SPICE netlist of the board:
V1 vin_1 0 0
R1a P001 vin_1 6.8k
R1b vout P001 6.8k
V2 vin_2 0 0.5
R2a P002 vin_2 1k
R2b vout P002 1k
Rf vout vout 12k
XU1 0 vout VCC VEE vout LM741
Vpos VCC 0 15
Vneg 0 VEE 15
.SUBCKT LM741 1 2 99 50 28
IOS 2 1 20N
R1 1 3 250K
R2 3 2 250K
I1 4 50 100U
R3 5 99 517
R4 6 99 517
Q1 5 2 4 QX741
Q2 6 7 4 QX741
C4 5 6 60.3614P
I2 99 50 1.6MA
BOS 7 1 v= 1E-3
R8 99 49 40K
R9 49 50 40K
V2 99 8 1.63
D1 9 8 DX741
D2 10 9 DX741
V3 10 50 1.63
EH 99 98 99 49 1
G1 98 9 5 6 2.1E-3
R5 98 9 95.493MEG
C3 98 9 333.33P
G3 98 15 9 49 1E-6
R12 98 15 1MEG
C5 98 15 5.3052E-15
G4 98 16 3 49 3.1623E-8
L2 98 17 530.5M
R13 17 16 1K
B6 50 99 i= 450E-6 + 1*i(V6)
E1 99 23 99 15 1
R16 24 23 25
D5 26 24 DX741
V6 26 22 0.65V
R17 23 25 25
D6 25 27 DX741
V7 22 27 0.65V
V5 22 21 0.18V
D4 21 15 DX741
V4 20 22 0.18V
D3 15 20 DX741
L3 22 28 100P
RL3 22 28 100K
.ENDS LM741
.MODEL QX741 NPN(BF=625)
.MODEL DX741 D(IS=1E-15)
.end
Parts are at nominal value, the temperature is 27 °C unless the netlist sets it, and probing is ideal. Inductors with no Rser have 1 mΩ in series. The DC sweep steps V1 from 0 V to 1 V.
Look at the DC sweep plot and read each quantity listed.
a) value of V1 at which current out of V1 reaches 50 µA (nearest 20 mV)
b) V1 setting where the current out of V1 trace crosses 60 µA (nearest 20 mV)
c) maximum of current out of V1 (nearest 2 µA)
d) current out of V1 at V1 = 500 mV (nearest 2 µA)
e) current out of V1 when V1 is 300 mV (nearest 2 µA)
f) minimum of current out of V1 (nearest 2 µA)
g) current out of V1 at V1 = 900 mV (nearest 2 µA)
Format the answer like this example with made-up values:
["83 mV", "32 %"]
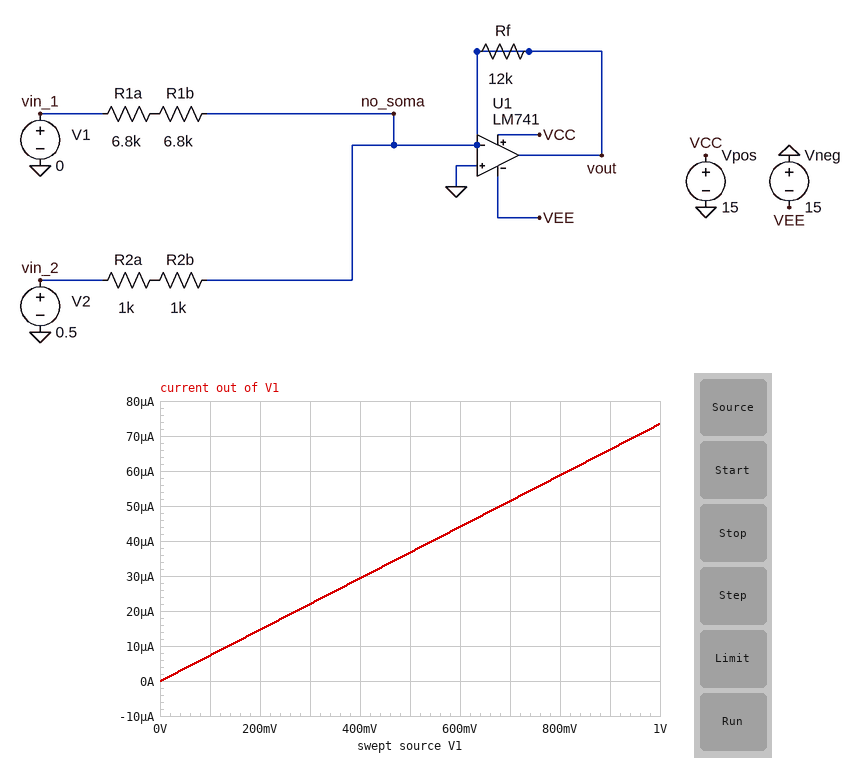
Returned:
["680 mV", "820 mV", "74 µA", "36 µA", "22 µA", "0 A", "66 µA"]
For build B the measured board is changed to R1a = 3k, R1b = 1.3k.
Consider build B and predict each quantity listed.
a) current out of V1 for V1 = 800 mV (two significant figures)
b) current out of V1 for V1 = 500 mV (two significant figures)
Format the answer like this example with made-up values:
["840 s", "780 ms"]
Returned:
["190 µA", "120 µA"]
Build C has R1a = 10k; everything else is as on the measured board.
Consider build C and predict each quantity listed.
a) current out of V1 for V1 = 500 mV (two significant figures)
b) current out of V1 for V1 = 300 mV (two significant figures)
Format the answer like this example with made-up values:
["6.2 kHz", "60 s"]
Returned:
["30 µA", "18 µA"]
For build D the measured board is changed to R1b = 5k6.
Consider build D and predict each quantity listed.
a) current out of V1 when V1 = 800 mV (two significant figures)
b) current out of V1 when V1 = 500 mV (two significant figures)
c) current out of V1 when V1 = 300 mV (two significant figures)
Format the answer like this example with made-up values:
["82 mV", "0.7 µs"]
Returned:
["64 µA", "40 µA", "24 µA"]
